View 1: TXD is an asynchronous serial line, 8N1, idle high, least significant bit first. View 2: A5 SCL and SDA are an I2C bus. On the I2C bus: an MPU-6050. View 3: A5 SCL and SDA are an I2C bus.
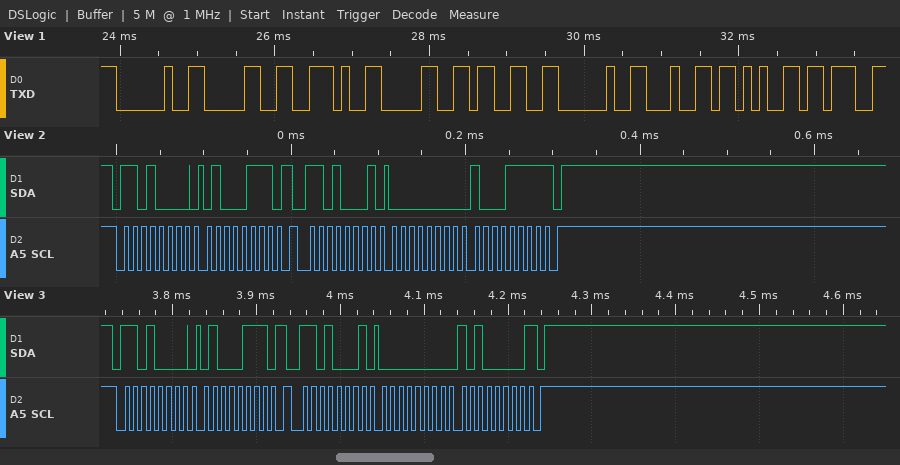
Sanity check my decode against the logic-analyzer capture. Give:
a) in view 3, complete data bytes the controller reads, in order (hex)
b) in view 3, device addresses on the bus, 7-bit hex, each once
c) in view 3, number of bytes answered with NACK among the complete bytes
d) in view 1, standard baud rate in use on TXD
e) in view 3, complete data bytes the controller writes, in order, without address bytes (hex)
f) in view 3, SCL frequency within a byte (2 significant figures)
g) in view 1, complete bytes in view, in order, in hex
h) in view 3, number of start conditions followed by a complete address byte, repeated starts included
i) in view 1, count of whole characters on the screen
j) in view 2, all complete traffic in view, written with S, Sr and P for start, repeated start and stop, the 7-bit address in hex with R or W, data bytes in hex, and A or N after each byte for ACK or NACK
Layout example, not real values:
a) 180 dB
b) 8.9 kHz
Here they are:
a) 00 A0
b) 0x68
c) 1
d) 9600 baud
e) 47
f) 100 kHz
g) 0x20 0x30 0x2E 0x30 0x33 0x20 0x64 0x65
h) 2
i) 8
j) S 68W A 47 A Sr 68R A 00 A 8F N P
